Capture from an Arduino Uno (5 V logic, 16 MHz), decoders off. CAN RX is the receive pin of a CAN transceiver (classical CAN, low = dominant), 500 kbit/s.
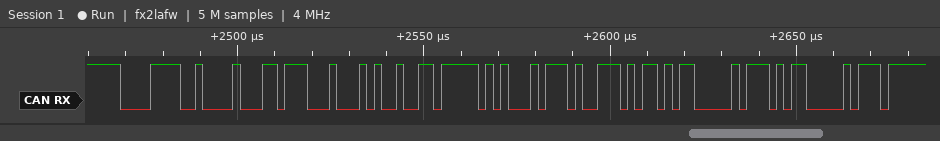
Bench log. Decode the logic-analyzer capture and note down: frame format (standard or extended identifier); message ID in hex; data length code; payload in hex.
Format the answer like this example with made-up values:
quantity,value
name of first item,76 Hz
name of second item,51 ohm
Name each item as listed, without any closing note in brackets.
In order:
quantity,value
frame format,standard
message ID in hex,0x0F2
data length code,8
payload in hex,DC 45 26 FD 17 4E B5 81
